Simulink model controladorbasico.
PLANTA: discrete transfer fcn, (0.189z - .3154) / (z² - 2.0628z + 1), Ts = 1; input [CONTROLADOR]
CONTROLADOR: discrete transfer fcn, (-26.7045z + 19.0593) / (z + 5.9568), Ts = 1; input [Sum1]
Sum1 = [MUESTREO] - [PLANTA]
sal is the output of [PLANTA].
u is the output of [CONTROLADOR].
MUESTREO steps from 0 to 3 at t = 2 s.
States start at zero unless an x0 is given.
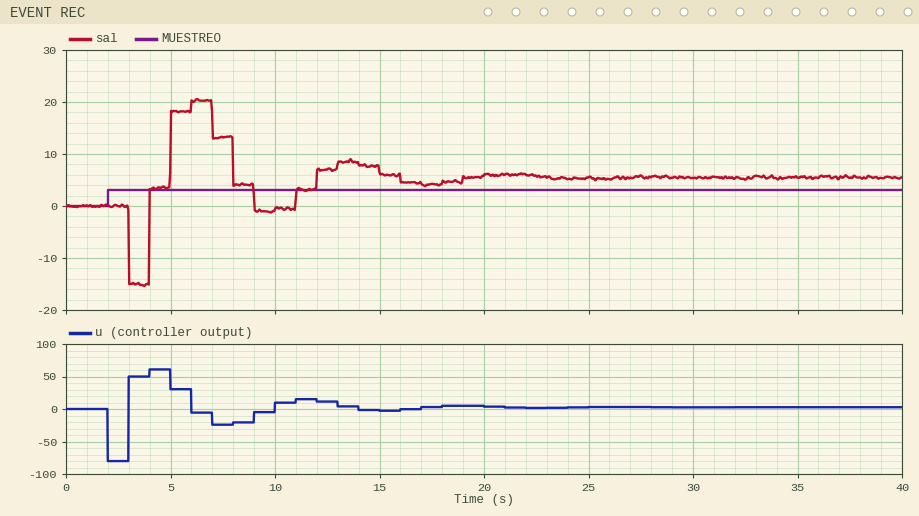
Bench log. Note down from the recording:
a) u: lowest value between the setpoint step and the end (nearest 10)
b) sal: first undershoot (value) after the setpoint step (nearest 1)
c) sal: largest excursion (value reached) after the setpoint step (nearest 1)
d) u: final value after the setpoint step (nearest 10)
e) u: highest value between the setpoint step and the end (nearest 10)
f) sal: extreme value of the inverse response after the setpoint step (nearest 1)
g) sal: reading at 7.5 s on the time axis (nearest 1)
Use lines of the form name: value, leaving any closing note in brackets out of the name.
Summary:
u: lowest value between the setpoint step and the end: -80
sal: first undershoot (value) after the setpoint step: -1
sal: largest excursion (value reached) after the setpoint step: 20
u: final value after the setpoint step: 0
u: highest value between the setpoint step and the end: 60
sal: extreme value of the inverse response after the setpoint step: -15
sal: reading at 7.5 s on the time axis: 13
